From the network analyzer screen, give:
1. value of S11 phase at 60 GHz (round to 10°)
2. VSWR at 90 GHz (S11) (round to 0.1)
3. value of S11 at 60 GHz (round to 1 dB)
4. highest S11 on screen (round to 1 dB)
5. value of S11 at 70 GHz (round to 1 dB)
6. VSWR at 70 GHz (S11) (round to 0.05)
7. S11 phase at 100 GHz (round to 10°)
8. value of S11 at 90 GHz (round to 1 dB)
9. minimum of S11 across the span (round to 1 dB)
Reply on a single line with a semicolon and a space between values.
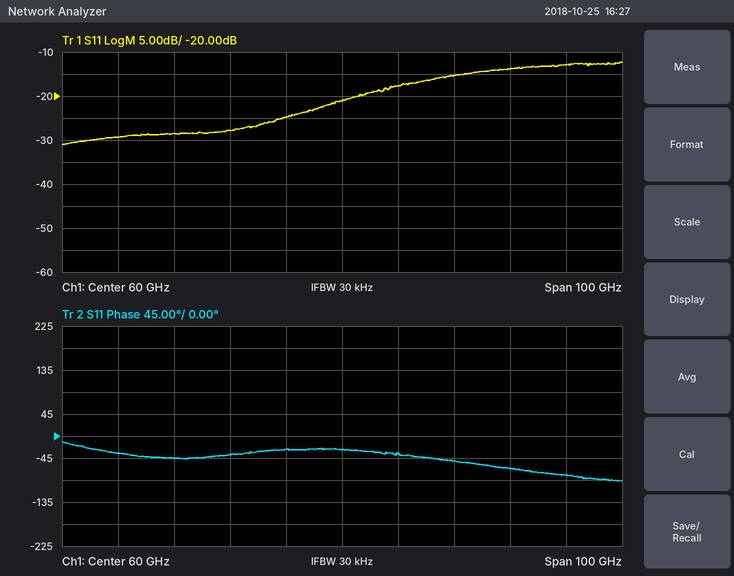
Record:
-30°; 1.5; -21 dB; -12 dB; -18 dB; 1.30; -80°; -14 dB; -31 dB
